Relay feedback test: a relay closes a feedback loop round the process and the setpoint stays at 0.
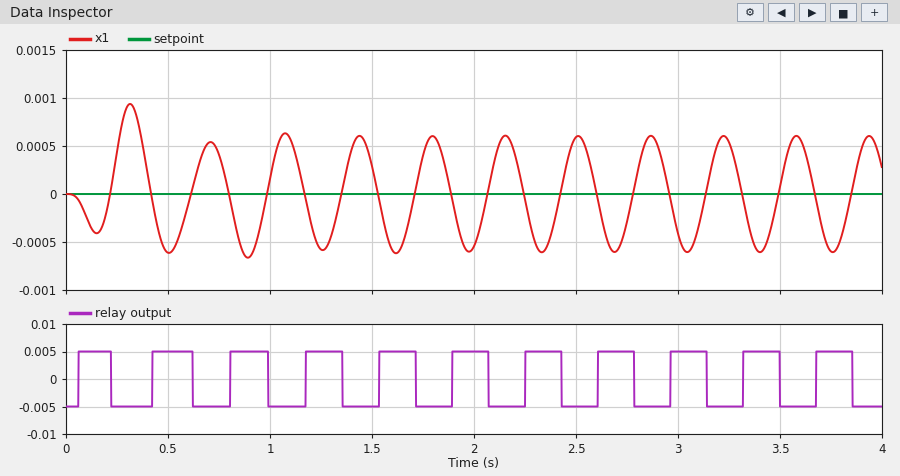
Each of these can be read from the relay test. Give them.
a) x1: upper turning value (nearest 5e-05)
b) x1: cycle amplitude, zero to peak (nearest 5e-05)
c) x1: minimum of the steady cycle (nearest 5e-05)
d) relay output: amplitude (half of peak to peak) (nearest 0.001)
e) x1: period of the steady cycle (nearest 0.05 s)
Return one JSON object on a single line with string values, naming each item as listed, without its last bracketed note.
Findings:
{"x1: upper turning value": "0.00060", "x1: cycle amplitude, zero to peak": "0.00060", "x1: minimum of the steady cycle": "-0.00060", "relay output: amplitude (half of peak to peak)": "0.005", "x1: period of the steady cycle": "0.35 s"}
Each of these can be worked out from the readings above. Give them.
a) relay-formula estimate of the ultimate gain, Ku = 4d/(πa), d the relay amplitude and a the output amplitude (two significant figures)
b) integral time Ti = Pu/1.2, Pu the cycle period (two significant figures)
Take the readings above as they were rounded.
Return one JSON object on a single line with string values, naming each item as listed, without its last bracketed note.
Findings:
{"relay-formula estimate of the ultimate gain, Ku = 4d/(πa), d the relay amplitude and a the output amplitude": "11", "integral time Ti = Pu/1.2, Pu the cycle period": "0.29 s"}
